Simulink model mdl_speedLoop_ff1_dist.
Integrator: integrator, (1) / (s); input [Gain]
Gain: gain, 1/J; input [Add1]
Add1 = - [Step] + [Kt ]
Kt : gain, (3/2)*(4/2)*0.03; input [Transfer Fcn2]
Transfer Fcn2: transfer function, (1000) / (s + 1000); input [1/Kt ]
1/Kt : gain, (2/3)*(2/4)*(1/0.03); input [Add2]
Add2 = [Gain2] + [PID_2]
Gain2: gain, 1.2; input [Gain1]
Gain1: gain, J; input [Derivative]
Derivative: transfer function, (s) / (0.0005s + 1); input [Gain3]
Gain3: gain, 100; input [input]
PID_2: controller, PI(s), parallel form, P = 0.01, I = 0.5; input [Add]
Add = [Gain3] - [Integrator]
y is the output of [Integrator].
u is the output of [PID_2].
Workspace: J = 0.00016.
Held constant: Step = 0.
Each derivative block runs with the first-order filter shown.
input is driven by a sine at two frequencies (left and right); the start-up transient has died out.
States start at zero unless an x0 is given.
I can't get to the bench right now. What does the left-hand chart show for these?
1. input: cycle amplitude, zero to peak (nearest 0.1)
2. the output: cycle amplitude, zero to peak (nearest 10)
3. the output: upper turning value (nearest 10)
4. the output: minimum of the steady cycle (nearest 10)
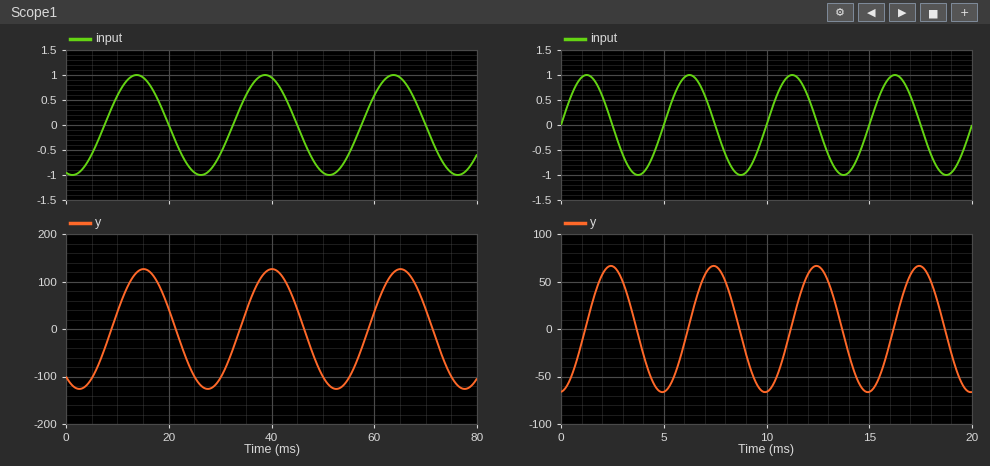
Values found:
1.0
130
130
-130
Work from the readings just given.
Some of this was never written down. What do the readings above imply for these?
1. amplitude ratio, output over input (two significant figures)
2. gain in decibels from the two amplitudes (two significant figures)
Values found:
130
42 dB
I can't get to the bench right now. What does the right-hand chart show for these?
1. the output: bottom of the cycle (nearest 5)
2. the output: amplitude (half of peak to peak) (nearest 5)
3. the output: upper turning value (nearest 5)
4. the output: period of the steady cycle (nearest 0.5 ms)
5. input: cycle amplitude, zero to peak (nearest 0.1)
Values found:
-65
65
65
5.0 ms
1.0
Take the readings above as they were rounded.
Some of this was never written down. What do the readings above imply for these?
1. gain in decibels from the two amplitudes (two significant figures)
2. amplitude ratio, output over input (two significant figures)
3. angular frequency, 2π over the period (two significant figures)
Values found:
36 dB
65
1.3 rad/ms
